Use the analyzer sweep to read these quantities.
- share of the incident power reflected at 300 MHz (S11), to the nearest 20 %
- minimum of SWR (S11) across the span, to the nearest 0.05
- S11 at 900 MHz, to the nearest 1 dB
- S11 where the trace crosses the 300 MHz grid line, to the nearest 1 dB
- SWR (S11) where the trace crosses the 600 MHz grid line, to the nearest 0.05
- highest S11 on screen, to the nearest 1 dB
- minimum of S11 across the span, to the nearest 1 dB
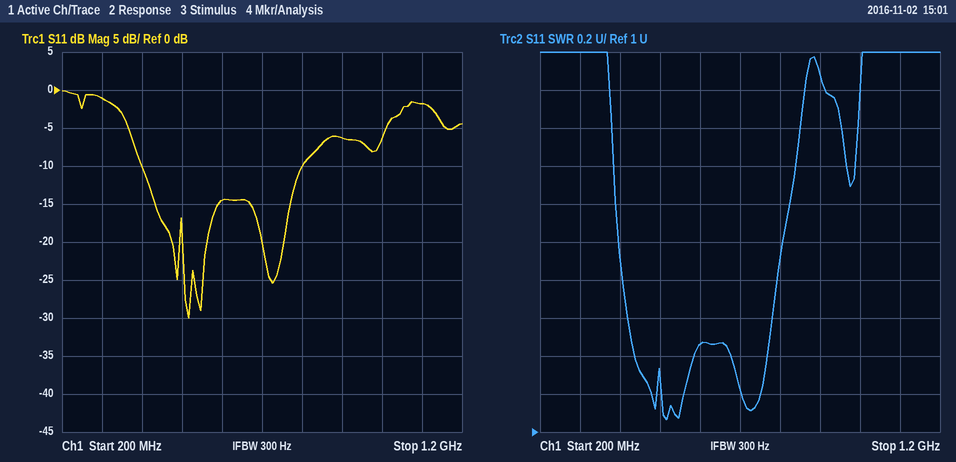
80 %
1.05
-6 dB
-1 dB
1.45
0 dB
-30 dB
